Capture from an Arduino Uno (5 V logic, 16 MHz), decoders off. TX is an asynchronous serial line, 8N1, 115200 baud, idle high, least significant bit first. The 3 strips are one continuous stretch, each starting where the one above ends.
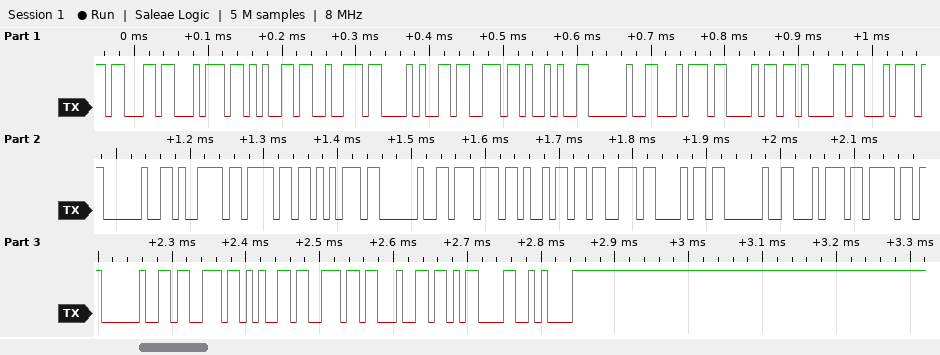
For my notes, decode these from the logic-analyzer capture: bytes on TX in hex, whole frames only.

63 74 65 72 28 73 29 20 74 68 61 74 20 79 6F 75 20 77 69 73 68 20 74 6F 20 73 65 6E 64 0D 0A
